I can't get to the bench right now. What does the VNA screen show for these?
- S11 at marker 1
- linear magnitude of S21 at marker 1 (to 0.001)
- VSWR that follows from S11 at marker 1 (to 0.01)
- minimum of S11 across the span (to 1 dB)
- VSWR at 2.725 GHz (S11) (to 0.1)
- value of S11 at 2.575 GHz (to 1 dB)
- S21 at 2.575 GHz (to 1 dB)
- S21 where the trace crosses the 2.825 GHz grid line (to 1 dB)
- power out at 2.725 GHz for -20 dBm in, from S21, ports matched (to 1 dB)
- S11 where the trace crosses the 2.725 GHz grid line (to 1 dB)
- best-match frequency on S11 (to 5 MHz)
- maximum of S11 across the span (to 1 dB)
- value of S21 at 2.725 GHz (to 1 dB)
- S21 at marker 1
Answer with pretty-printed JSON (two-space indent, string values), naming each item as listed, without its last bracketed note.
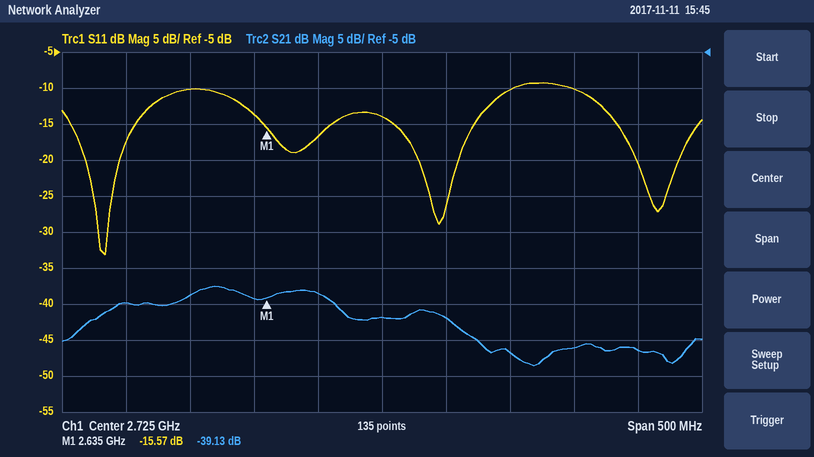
{
  "S11 at marker 1": "-15.57 dB",
  "linear magnitude of S21 at marker 1": "0.011",
  "VSWR that follows from S11 at marker 1": "1.40",
  "minimum of S11 across the span": "-33 dB",
  "VSWR at 2.725 GHz (S11)": "1.5",
  "value of S11 at 2.575 GHz": "-10 dB",
  "S21 at 2.575 GHz": "-39 dB",
  "S21 where the trace crosses the 2.825 GHz grid line": "-47 dB",
  "power out at 2.725 GHz for -20 dBm in, from S21, ports matched": "-62 dBm",
  "S11 where the trace crosses the 2.725 GHz grid line": "-14 dB",
  "best-match frequency on S11": "2.510 GHz",
  "maximum of S11 across the span": "-9 dB",
  "value of S21 at 2.725 GHz": "-42 dB",
  "S21 at marker 1": "-39.13 dB"
}
